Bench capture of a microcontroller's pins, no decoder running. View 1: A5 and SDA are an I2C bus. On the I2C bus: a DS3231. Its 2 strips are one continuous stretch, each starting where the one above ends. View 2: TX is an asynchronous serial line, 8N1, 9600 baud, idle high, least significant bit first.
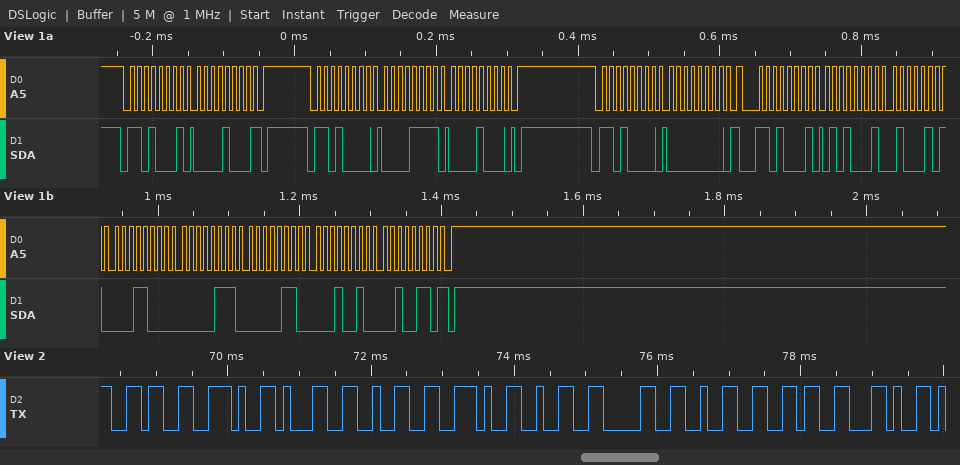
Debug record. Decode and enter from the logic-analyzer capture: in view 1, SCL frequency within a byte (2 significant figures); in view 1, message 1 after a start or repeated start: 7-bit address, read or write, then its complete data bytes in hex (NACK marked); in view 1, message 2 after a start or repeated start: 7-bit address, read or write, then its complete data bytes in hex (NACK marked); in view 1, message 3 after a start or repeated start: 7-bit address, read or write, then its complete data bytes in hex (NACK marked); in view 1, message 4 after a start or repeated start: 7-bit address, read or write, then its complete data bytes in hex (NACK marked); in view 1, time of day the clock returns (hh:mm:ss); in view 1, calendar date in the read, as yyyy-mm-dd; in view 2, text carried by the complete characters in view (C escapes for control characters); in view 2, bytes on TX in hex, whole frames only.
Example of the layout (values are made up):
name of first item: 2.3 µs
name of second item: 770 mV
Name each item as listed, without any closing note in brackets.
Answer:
in view 1, SCL frequency within a byte: 100 kHz
in view 1, message 1 after a start or repeated start: 7-bit address, read or write, then its complete data bytes in hex: 0x68 read: 08 NACK
in view 1, message 2 after a start or repeated start: 7-bit address, read or write, then its complete data bytes in hex: 0x68 write: 0F 08
in view 1, message 3 after a start or repeated start: 7-bit address, read or write, then its complete data bytes in hex: 0x68 write: 00
in view 1, message 4 after a start or repeated start: 7-bit address, read or write, then its complete data bytes in hex: 0x68 read: 51 45 18 07 06 12 26 NACK
in view 1, time of day the clock returns: 18:45:51
in view 1, calendar date in the read, as yyyy-mm-dd: 2026-12-06
in view 2, text carried by the complete characters in view: "6.12.2026,"
in view 2, bytes on TX in hex, whole frames only: 36 2E 31 32 2E 32 30 32 36 2C
